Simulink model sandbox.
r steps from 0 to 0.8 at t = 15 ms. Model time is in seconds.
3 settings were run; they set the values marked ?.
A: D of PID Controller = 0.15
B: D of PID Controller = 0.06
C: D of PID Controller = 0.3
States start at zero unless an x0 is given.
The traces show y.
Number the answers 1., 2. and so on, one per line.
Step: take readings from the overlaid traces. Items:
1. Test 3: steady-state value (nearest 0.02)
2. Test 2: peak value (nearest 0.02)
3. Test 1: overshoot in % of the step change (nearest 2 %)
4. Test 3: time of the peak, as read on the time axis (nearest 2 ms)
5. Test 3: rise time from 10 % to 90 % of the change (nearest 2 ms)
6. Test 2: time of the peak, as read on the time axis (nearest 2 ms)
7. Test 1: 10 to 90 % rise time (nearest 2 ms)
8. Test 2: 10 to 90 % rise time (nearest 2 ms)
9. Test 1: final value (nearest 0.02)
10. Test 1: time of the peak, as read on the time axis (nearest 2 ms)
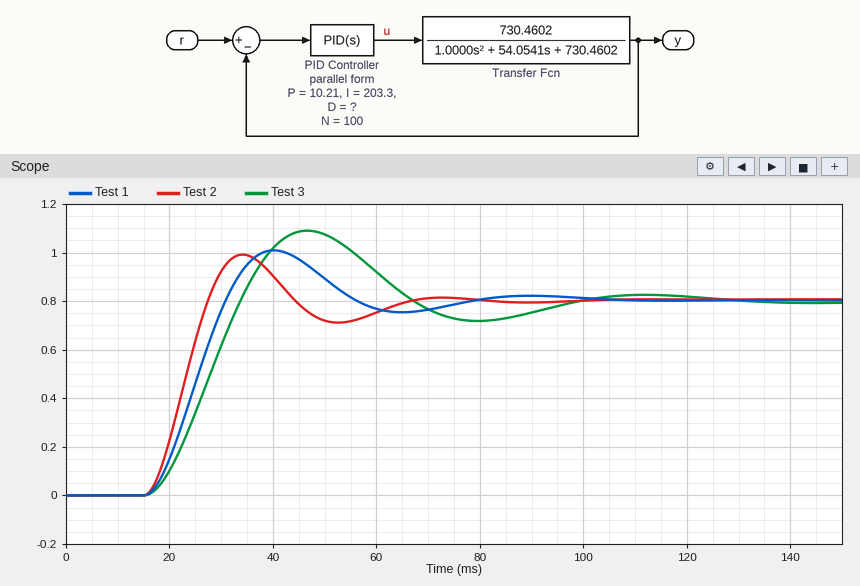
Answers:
1. 0.80
2. 1.00
3. 26 %
4. 46 ms
5. 12 ms
6. 34 ms
7. 10 ms
8. 8 ms
9. 0.80
10. 40 ms
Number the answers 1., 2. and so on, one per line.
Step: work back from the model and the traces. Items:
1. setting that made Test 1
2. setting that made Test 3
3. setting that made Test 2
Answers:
1. A
2. B
3. C
